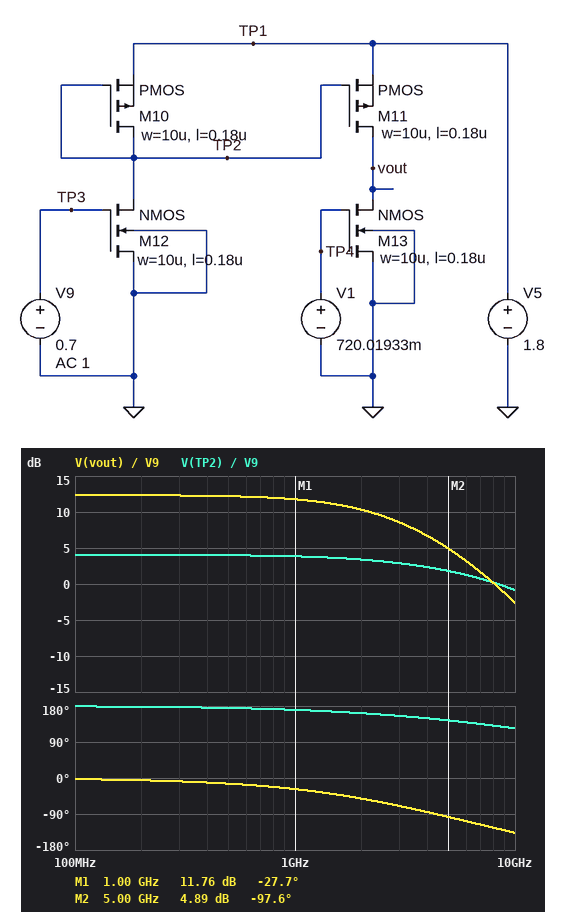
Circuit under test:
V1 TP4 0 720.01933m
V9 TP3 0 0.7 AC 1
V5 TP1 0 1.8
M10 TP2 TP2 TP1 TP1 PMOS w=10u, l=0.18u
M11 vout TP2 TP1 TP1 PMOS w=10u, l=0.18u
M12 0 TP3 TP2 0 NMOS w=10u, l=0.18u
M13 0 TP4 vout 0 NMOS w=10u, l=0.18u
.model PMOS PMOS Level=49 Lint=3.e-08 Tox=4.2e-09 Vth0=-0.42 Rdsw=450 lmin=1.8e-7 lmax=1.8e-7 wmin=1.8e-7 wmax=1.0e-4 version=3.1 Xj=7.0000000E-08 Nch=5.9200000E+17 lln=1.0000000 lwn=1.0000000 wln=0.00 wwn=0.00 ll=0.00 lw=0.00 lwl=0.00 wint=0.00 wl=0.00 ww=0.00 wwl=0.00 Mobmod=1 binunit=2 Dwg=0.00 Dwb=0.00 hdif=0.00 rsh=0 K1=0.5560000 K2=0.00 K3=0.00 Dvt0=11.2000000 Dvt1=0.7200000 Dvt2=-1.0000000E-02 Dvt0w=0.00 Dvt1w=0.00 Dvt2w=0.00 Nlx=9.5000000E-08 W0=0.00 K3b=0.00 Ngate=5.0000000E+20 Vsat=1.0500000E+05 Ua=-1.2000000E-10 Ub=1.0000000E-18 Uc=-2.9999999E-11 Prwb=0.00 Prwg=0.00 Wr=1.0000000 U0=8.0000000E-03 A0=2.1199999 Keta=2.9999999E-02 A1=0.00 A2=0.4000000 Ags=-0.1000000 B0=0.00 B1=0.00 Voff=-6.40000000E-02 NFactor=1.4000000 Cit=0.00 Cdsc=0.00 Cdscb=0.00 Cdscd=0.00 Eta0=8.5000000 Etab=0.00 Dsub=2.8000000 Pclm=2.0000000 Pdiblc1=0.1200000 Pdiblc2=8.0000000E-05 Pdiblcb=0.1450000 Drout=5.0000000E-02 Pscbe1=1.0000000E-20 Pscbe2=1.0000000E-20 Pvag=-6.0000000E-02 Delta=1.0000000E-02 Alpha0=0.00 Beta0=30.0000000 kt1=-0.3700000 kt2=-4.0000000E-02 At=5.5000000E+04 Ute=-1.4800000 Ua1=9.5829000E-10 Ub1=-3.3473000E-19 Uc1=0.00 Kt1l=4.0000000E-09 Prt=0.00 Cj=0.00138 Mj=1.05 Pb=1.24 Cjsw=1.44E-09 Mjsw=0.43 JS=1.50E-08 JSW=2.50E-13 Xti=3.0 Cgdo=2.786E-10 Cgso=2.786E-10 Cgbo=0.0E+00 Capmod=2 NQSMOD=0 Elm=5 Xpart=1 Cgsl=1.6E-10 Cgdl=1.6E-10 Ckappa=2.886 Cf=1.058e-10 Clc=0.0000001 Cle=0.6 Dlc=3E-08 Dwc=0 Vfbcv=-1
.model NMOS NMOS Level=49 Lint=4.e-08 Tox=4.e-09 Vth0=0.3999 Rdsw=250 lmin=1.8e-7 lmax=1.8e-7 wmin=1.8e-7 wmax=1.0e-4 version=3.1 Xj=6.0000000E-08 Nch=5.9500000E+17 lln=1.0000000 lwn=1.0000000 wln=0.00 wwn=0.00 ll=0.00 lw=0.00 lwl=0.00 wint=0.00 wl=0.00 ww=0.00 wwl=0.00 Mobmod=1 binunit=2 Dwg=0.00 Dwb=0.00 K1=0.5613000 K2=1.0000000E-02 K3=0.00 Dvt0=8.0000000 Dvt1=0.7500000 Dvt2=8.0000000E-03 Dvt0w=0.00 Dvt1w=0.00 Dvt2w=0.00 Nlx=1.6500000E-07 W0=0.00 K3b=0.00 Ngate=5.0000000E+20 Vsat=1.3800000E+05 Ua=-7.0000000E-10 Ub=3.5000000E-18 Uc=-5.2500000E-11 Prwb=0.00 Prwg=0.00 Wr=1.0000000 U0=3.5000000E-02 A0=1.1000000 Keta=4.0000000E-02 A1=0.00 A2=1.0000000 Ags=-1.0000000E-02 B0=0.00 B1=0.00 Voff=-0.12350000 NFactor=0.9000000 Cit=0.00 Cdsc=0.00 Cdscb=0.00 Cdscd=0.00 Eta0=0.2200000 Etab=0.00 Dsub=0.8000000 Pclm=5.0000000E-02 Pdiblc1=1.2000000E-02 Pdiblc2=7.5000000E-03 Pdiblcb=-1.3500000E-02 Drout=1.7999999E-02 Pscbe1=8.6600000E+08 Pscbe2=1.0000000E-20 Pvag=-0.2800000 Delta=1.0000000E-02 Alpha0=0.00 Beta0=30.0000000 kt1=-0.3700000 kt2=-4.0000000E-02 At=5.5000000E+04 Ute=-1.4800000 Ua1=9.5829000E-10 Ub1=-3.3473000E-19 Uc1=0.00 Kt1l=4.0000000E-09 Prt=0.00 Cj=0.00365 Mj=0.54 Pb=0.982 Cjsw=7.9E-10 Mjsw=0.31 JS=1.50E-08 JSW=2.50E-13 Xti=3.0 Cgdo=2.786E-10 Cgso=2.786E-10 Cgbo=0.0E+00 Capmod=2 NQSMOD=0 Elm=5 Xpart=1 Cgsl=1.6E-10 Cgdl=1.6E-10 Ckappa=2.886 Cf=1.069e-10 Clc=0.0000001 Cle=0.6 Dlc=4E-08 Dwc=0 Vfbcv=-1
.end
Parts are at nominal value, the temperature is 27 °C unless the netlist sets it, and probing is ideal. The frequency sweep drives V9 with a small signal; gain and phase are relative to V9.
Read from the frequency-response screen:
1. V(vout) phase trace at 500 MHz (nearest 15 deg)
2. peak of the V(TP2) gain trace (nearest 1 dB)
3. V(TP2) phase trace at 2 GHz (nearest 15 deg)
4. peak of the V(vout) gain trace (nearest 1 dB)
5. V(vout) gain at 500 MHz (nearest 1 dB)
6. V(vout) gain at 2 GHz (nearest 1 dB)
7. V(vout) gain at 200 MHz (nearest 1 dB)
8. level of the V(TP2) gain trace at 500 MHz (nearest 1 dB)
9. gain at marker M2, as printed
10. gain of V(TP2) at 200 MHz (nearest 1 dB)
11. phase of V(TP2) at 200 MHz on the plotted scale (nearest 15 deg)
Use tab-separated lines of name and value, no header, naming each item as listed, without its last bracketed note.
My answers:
V(vout) phase trace at 500 MHz	-15 deg
peak of the V(TP2) gain trace	4 dB
V(TP2) phase trace at 2 GHz	165 deg
peak of the V(vout) gain trace	12 dB
V(vout) gain at 500 MHz	12 dB
V(vout) gain at 2 GHz	10 dB
V(vout) gain at 200 MHz	12 dB
level of the V(TP2) gain trace at 500 MHz	4 dB
gain at marker M2, as printed	4.89 dB
gain of V(TP2) at 200 MHz	4 dB
phase of V(TP2) at 200 MHz on the plotted scale	180 deg
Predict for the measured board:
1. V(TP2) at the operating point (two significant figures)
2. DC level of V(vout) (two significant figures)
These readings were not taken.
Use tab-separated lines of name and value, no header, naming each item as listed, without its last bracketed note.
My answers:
V(TP2) at the operating point	850 mV
DC level of V(vout)	740 mV
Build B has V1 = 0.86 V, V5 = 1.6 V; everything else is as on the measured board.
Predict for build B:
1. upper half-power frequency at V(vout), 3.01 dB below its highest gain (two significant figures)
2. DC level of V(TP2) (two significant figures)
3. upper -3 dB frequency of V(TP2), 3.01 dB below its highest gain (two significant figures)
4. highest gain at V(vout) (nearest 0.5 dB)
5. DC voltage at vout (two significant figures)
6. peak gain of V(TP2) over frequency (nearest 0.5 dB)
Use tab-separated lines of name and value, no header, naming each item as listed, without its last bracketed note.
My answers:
upper half-power frequency at V(vout), 3.01 dB below its highest gain	5.9 GHz
DC level of V(TP2)	680 mV
upper -3 dB frequency of V(TP2), 3.01 dB below its highest gain	6.8 GHz
highest gain at V(vout)	-1.5 dB
DC voltage at vout	180 mV
peak gain of V(TP2) over frequency	4.0 dB
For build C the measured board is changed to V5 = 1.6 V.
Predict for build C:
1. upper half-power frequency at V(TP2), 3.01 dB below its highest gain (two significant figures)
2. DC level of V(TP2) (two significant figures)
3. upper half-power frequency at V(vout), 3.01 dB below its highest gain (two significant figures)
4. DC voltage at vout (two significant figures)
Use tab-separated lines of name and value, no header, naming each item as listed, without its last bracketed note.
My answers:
upper half-power frequency at V(TP2), 3.01 dB below its highest gain	6.3 GHz
DC level of V(TP2)	680 mV
upper half-power frequency at V(vout), 3.01 dB below its highest gain	2.5 GHz
DC voltage at vout	570 mV
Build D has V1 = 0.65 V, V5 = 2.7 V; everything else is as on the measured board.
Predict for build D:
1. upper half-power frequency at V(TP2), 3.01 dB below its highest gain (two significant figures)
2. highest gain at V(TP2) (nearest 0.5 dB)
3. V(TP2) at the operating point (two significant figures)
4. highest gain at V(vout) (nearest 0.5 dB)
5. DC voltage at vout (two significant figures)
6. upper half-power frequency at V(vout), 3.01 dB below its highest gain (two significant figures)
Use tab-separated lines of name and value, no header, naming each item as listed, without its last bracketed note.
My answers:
upper half-power frequency at V(TP2), 3.01 dB below its highest gain	7.3 GHz
highest gain at V(TP2)	4.5 dB
V(TP2) at the operating point	1.6 V
highest gain at V(vout)	10.5 dB
DC voltage at vout	1.9 V
upper half-power frequency at V(vout), 3.01 dB below its highest gain	3.1 GHz
